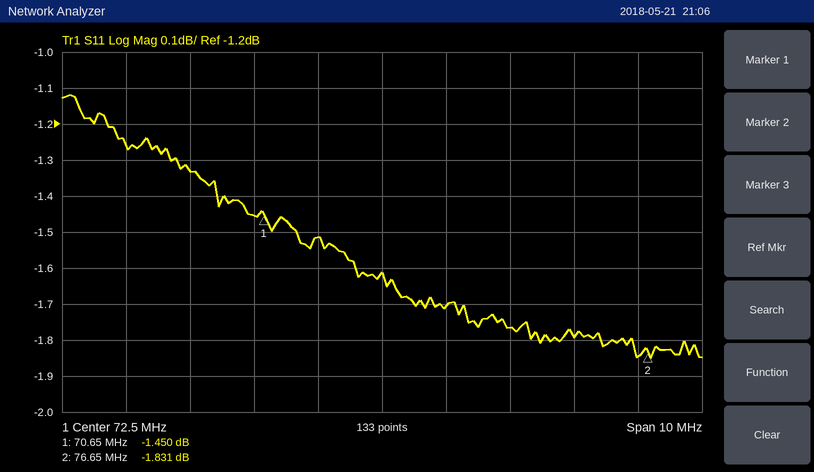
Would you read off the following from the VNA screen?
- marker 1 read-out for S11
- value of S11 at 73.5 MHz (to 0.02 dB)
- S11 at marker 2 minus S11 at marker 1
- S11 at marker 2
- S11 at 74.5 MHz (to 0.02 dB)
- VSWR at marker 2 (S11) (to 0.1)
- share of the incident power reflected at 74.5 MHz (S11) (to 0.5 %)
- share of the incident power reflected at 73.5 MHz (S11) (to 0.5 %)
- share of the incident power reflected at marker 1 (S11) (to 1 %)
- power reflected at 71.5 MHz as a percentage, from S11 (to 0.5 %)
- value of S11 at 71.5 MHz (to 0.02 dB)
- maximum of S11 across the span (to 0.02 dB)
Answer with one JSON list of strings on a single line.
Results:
["-1.450 dB", "-1.70 dB", "-0.381 dB", "-1.831 dB", "-1.76 dB", "9.5", "66.5 %", "67.5 %", "72 %", "70.5 %", "-1.52 dB", "-1.12 dB"]
